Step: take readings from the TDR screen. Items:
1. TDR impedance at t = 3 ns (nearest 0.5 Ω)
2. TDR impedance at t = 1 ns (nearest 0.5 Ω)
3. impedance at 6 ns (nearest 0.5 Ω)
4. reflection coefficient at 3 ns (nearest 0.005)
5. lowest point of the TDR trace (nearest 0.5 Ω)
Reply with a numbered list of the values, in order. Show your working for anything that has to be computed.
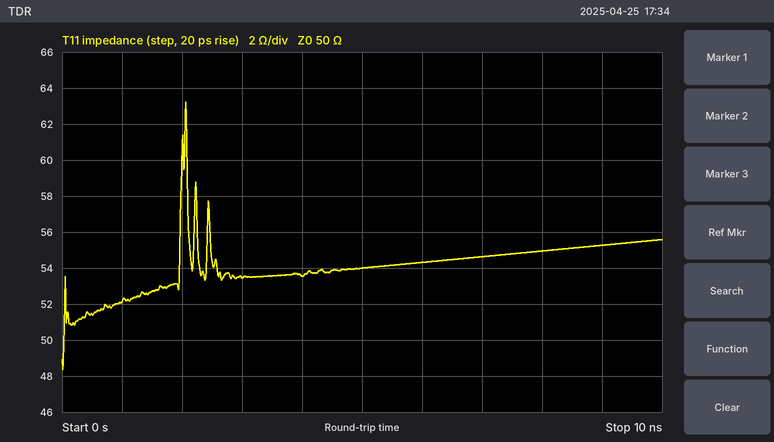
1. 53.5 Ω
2. 52.0 Ω
3. 54.5 Ω
4. (53.5 − 50)/(53.5 + 50) ≈ +0.0338, so +0.035 to the nearest 0.005
5. 48.5 Ω
